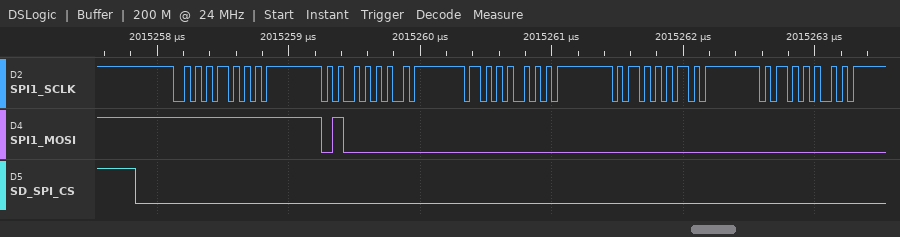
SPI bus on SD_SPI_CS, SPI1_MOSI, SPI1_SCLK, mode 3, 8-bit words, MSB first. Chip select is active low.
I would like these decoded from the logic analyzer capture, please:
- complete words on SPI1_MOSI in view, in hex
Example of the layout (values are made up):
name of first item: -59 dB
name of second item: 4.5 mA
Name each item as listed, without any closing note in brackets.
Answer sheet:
complete words on SPI1_MOSI in view, in hex: FF, 40, 00, 00, 00
